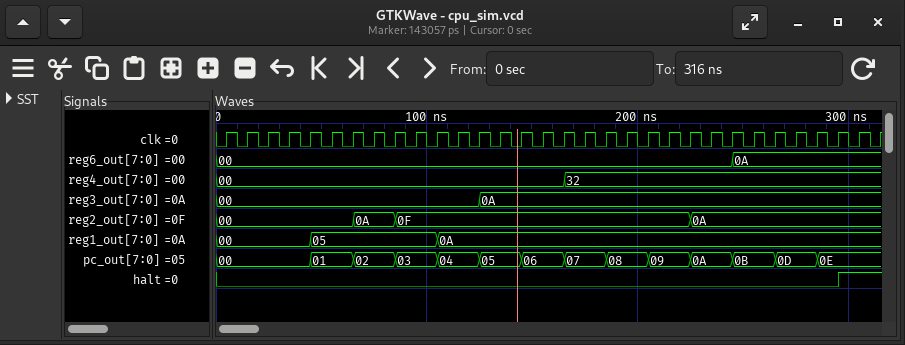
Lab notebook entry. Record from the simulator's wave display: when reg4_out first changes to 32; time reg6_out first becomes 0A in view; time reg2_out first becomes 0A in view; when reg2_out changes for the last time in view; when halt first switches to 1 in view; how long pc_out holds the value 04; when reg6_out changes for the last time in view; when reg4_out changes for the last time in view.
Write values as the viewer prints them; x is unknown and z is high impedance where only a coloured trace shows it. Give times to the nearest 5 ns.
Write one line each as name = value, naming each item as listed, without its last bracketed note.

when reg4_out first changes to 32 = 165 ns
time reg6_out first becomes 0A in view = 245 ns
time reg2_out first becomes 0A in view = 65 ns
when reg2_out changes for the last time in view = 225 ns
when halt first switches to 1 in view = 295 ns
how long pc_out holds the value 04 = 20 ns
when reg6_out changes for the last time in view = 245 ns
when reg4_out changes for the last time in view = 165 ns
